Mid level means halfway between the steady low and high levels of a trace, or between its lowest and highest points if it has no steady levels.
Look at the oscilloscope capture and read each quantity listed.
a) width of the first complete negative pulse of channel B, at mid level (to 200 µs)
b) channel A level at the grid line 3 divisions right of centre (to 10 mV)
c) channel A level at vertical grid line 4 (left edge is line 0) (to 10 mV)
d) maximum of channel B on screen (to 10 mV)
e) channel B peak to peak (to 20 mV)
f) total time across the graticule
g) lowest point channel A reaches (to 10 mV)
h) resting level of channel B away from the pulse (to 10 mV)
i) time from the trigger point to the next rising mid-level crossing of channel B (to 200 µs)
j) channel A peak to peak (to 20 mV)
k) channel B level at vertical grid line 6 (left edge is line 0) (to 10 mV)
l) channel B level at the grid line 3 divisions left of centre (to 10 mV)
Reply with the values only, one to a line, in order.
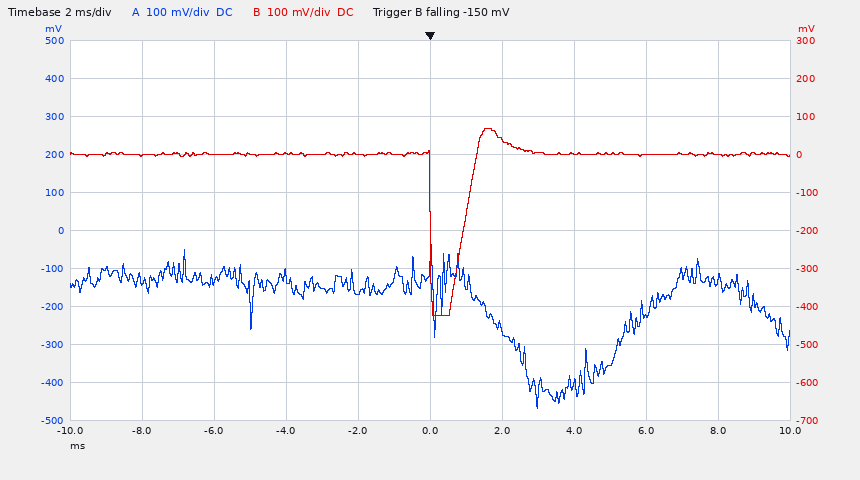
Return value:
1.0 ms
-220 mV
-160 mV
70 mV
500 mV
20 ms
-470 mV
0 mV
1.0 ms
440 mV
40 mV
0 mV
